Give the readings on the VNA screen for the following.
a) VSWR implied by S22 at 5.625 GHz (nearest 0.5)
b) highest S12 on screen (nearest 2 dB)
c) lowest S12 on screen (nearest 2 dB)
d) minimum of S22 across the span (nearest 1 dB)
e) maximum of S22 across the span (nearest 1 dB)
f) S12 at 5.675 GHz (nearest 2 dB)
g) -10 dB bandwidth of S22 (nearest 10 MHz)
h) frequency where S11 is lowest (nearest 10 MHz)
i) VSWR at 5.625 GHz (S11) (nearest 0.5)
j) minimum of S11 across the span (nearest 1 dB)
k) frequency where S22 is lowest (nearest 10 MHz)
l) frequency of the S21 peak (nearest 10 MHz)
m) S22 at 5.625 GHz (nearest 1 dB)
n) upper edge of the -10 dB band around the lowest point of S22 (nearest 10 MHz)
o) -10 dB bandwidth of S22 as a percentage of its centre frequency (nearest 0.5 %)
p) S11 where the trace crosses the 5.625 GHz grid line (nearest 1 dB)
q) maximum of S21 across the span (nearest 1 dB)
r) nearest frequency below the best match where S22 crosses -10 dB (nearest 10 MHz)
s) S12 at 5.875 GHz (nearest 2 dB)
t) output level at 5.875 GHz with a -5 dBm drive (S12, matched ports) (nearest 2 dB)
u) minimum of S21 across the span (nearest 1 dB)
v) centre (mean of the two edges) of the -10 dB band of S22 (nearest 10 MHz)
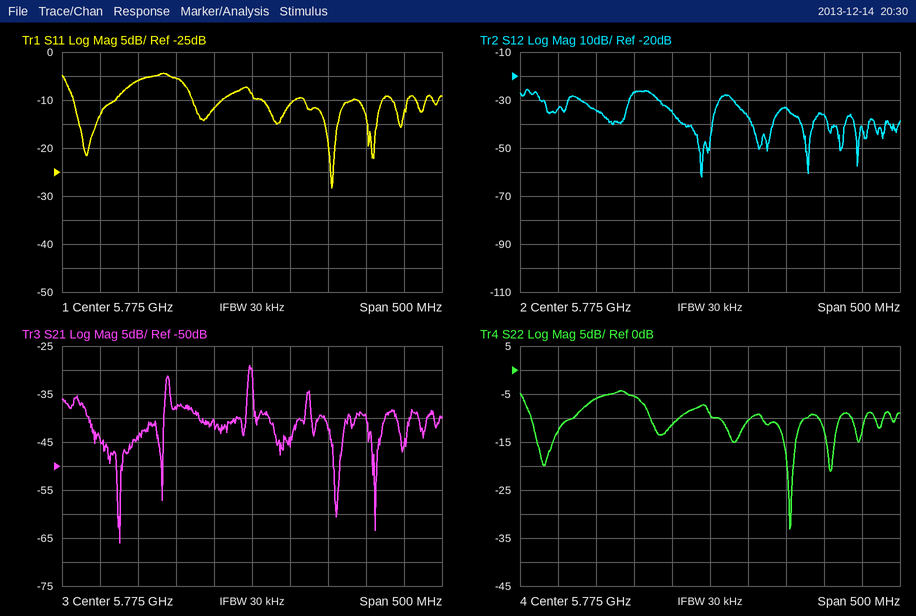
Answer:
3.0
-26 dB
-62 dB
-33 dB
-4 dB
-26 dB
60 MHz
5.88 GHz
3.0
-28 dB
5.88 GHz
5.77 GHz
-6 dB
5.90 GHz
1.0 %
-6 dB
-29 dB
5.84 GHz
-34 dB
-38 dBm
-66 dB
5.87 GHz
